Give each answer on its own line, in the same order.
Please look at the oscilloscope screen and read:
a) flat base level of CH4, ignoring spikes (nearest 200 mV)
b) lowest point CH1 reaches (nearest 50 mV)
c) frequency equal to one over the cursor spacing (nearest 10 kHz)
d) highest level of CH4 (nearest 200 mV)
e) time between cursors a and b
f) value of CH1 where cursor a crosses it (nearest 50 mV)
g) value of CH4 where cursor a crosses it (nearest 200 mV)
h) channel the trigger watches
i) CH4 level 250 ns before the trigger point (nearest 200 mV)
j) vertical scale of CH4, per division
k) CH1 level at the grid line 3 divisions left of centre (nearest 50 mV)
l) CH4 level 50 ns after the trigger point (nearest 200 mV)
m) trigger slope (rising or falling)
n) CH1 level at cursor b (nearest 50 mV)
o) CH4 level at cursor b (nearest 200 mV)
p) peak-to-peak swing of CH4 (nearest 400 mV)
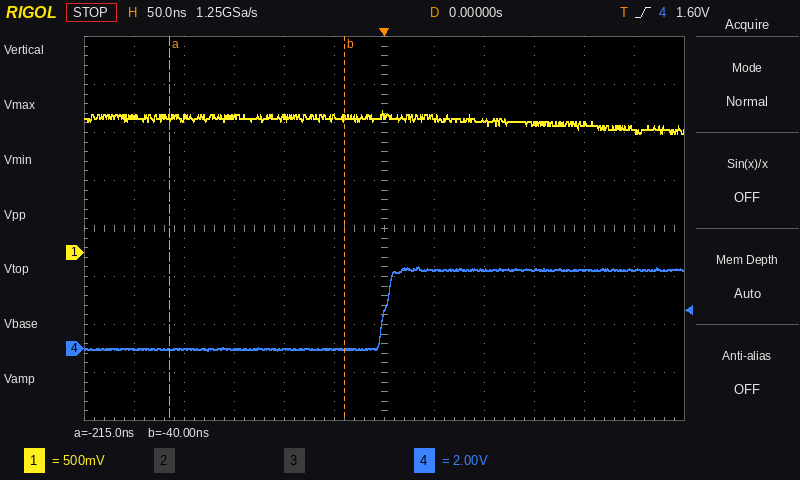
0.0 V
1.25 V
5.71 MHz
3.4 V
175 ns
1.40 V
0.0 V
CH4
0.0 V
2 V
1.40 V
3.2 V
rising
1.40 V
0.0 V
3.6 V
